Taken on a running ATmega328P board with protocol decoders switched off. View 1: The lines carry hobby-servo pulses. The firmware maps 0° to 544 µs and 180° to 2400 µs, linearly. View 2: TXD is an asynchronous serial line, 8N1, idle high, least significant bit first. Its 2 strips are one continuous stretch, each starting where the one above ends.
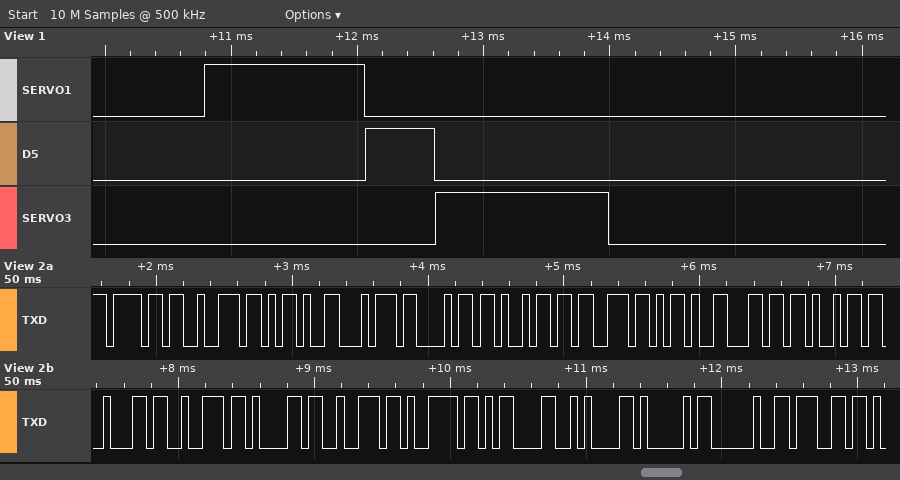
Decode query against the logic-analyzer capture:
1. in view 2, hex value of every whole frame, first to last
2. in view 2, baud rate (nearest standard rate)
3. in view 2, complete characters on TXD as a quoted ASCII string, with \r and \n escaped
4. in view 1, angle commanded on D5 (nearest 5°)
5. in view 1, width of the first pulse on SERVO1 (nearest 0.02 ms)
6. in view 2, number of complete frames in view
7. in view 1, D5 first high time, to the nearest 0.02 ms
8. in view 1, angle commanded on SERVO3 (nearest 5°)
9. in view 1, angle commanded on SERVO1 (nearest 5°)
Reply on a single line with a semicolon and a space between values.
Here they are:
6F 72 2D 74 68 69 73 2D 6C 69 62 72 61 72 79 0D 0A 41 20 67; 19200 baud; "or-this-library\r\nA g"; 0°; 1.26 ms; 20; 0.54 ms; 80°; 70°
